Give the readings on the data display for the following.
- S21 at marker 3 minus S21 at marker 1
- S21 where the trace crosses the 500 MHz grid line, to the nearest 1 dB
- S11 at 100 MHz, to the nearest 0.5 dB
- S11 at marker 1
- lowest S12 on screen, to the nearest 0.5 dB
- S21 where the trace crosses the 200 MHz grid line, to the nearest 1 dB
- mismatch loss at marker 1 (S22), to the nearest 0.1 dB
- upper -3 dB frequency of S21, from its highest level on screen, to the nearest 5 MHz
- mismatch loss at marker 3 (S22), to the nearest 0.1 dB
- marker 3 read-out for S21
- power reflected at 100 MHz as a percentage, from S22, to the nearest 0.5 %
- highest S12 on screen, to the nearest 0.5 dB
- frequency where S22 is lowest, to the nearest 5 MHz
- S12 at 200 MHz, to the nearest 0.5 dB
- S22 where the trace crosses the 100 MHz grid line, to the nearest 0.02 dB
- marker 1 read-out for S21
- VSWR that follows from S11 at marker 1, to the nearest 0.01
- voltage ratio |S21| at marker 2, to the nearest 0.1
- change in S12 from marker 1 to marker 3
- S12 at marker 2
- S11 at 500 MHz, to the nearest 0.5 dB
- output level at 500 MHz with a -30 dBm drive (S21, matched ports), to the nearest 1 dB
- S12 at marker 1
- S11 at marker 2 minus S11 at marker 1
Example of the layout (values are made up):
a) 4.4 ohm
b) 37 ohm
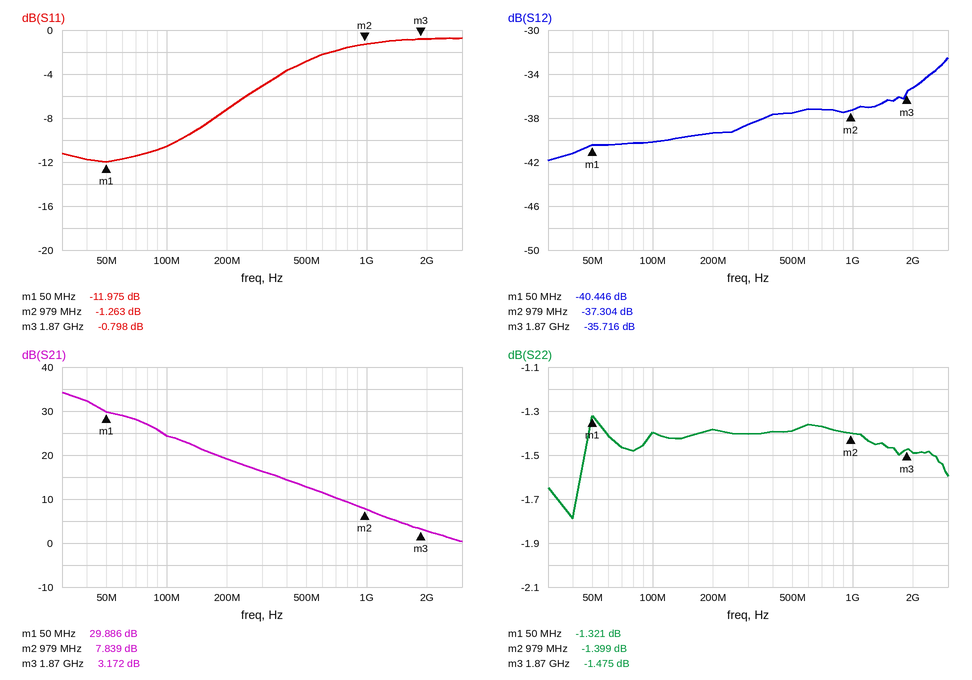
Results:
a) -26.714 dB
b) 13 dB
c) -10.5 dB
d) -11.975 dB
e) -42.0 dB
f) 19 dB
g) 5.8 dB
h) 45 MHz
i) 5.4 dB
j) 3.172 dB
k) 72.5 %
l) -32.5 dB
m) 40 MHz
n) -39.5 dB
o) -1.40 dB
p) 29.886 dB
q) 1.67
r) 2.5
s) 4.730 dB
t) -37.304 dB
u) -3.0 dB
v) -17 dBm
w) -40.446 dB
x) 10.712 dB
